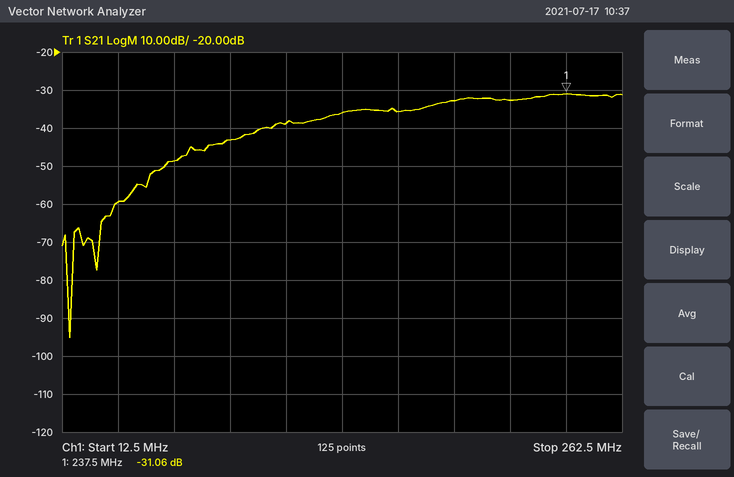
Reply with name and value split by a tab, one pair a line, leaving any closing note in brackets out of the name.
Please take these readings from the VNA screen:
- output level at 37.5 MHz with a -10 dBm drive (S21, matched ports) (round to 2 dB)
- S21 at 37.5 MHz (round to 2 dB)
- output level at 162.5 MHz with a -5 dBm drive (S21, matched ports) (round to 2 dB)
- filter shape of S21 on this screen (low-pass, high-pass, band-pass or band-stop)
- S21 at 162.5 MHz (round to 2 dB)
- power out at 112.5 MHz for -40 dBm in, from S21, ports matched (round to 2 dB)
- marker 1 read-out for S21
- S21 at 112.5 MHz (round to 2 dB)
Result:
output level at 37.5 MHz with a -10 dBm drive (S21, matched ports)	-70 dBm
S21 at 37.5 MHz	-60 dB
output level at 162.5 MHz with a -5 dBm drive (S21, matched ports)	-40 dBm
filter shape of S21 on this screen	high-pass
S21 at 162.5 MHz	-36 dB
power out at 112.5 MHz for -40 dBm in, from S21, ports matched	-78 dBm
marker 1 read-out for S21	-31.06 dB
S21 at 112.5 MHz	-38 dB
